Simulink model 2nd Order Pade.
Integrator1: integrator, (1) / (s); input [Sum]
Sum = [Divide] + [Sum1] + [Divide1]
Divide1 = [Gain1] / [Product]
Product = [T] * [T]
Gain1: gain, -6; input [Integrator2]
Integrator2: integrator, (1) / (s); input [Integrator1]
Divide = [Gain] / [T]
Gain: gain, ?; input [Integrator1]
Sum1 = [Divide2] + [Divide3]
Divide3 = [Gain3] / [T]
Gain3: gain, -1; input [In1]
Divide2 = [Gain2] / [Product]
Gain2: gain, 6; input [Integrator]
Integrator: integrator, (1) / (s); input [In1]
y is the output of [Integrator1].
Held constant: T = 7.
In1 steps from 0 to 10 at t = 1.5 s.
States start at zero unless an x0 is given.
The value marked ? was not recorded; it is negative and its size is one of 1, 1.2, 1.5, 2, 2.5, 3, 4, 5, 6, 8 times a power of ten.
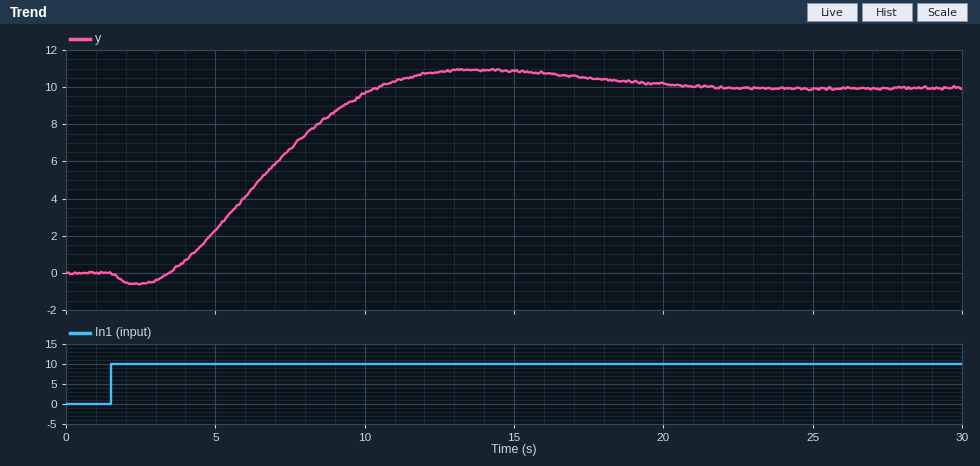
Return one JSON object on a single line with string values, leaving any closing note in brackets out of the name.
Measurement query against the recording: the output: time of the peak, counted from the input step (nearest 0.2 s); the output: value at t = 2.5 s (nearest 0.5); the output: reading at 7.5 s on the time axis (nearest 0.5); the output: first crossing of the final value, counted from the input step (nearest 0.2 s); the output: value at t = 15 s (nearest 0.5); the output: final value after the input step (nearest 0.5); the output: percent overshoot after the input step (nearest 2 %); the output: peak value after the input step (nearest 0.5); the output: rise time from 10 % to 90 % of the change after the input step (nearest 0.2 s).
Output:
{"the output: time of the peak, counted from the input step": "12.2 s", "the output: value at t = 2.5 s": "-0.5", "the output: reading at 7.5 s on the time axis": "6.5", "the output: first crossing of the final value, counted from the input step": "9.0 s", "the output: value at t = 15 s": "11.0", "the output: final value after the input step": "10.0", "the output: percent overshoot after the input step": "10 %", "the output: peak value after the input step": "11.0", "the output: rise time from 10 % to 90 % of the change after the input step": "5.0 s"}
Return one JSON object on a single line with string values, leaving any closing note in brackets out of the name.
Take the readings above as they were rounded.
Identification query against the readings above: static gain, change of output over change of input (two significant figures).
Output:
{"static gain, change of output over change of input": "1.0"}
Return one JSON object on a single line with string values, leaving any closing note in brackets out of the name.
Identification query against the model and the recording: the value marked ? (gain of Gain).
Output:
{"the value marked ?": "-3"}
